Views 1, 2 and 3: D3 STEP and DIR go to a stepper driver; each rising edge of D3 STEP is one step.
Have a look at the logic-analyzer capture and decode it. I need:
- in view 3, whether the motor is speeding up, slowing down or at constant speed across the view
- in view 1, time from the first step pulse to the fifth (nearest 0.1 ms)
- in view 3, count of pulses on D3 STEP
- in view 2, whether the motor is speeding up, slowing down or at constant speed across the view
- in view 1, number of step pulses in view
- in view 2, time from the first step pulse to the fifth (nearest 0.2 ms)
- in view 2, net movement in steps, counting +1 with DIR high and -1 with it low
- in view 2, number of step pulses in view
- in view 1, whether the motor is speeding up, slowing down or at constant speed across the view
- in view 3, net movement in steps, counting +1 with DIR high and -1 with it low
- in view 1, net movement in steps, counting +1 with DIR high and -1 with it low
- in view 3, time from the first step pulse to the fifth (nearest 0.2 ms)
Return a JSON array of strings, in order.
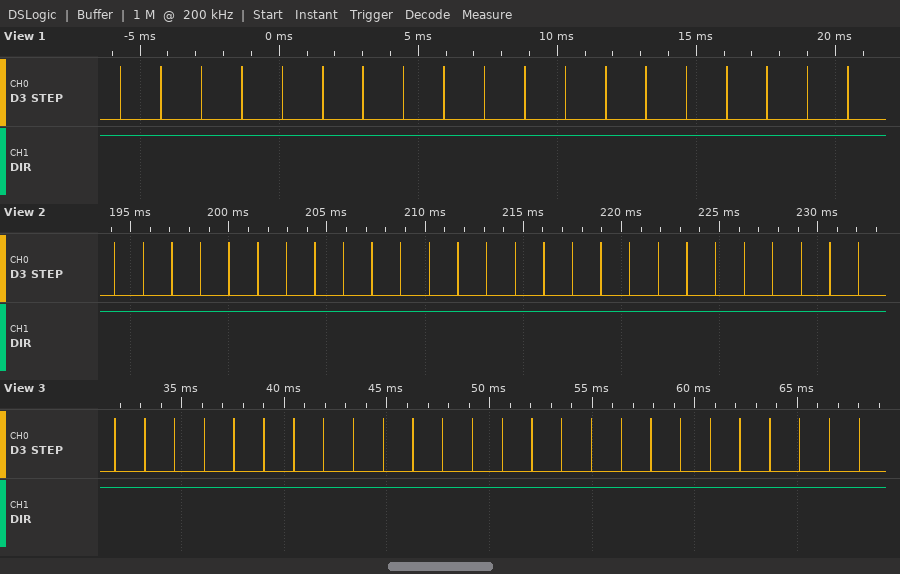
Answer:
["constant speed", "5.8 ms", "26", "constant speed", "19", "5.8 ms", "+27", "27", "constant speed", "+26", "+19", "5.8 ms"]
